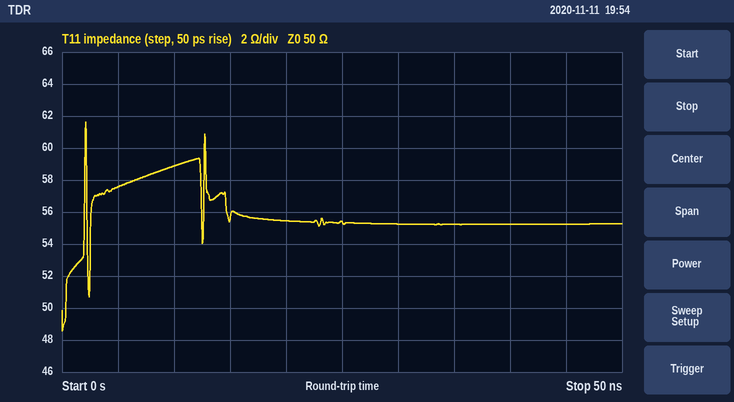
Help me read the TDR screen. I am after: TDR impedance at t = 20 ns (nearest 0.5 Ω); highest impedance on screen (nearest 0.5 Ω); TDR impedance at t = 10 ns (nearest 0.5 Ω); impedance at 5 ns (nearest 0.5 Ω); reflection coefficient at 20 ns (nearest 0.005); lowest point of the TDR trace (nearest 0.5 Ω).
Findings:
55.5 Ω
61.5 Ω
59.0 Ω
57.5 Ω
+0.050
48.5 Ω
